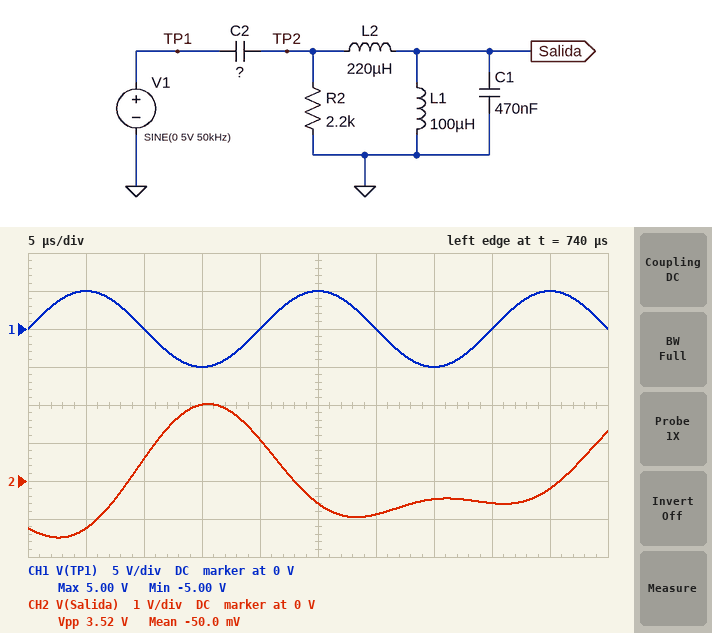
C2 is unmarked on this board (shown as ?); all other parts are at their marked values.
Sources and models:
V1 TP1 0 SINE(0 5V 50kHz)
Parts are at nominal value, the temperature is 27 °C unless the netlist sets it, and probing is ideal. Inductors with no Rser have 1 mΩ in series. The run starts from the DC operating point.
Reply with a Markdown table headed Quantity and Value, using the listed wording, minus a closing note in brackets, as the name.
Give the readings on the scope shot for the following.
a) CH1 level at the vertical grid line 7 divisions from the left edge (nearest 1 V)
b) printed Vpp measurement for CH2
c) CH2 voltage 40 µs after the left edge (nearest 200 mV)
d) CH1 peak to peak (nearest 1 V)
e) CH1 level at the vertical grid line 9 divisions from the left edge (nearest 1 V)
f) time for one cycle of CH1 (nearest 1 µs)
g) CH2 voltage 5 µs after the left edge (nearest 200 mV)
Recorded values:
| Quantity | Value |
|---|---|
| CH1 level at the vertical grid line 7 divisions from the left edge | -5 V |
| printed Vpp measurement for CH2 | 3.52 V |
| CH2 voltage 40 µs after the left edge | -600 mV |
| CH1 peak to peak | 10 V |
| CH1 level at the vertical grid line 9 divisions from the left edge | 5 V |
| time for one cycle of CH1 | 20 µs |
| CH2 voltage 5 µs after the left edge | -1.2 V |
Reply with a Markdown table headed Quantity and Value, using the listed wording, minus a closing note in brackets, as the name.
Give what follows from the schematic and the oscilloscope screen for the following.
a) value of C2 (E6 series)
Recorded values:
| Quantity | Value |
|---|---|
| value of C2 | 6.8 µF |
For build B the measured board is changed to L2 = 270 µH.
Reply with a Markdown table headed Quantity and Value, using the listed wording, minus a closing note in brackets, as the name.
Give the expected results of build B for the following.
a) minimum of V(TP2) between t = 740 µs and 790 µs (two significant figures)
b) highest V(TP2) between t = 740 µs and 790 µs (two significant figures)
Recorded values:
| Quantity | Value |
|---|---|
| minimum of V(TP2) between t = 740 µs and 790 µs | -5.2 V |
| highest V(TP2) between t = 740 µs and 790 µs | 5.0 V |
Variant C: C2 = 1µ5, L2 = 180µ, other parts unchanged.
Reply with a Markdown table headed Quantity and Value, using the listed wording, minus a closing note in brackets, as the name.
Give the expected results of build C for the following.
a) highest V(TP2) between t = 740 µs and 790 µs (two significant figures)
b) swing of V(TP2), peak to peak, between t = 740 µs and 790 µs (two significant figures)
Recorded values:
| Quantity | Value |
|---|---|
| highest V(TP2) between t = 740 µs and 790 µs | 6.0 V |
| swing of V(TP2), peak to peak, between t = 740 µs and 790 µs | 11 V |
